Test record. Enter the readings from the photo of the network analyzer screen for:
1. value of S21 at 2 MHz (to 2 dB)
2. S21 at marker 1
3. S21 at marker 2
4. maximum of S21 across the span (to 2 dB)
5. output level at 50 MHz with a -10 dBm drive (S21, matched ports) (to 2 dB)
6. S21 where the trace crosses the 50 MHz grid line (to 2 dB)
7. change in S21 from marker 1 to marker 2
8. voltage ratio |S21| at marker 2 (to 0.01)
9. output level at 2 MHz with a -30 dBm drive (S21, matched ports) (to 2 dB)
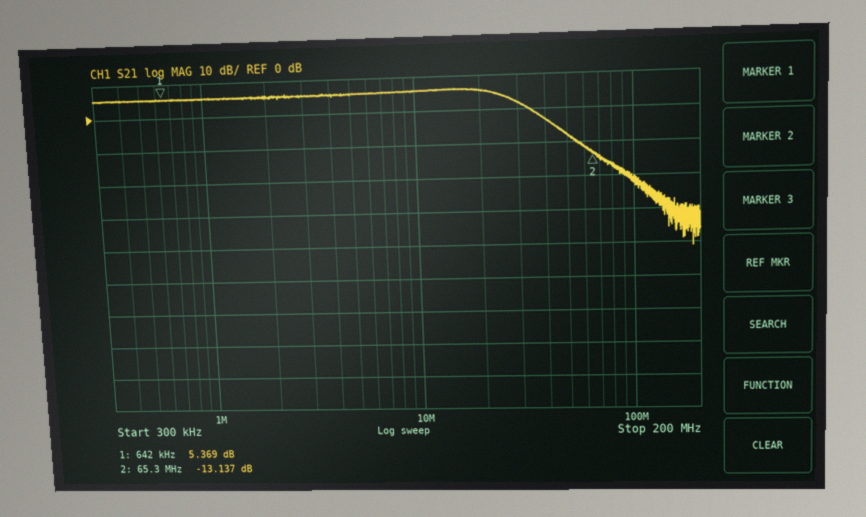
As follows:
6 dB
5.369 dB
-13.137 dB
6 dB
-18 dBm
-8 dB
-18.506 dB
0.22
-24 dBm
